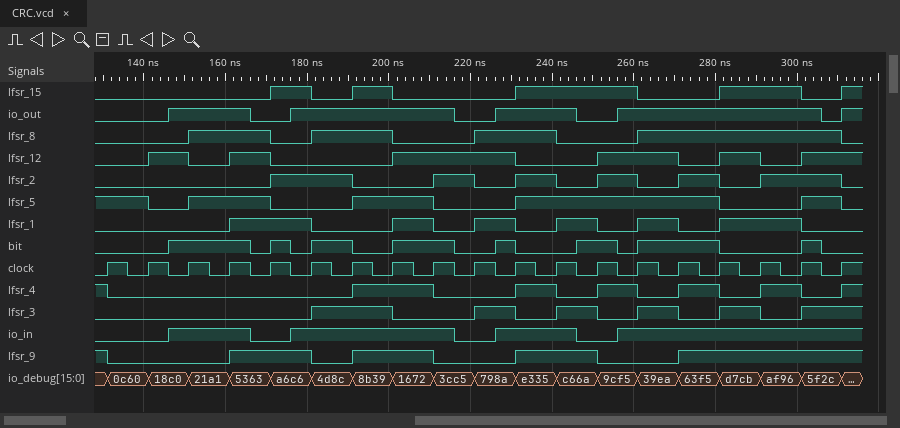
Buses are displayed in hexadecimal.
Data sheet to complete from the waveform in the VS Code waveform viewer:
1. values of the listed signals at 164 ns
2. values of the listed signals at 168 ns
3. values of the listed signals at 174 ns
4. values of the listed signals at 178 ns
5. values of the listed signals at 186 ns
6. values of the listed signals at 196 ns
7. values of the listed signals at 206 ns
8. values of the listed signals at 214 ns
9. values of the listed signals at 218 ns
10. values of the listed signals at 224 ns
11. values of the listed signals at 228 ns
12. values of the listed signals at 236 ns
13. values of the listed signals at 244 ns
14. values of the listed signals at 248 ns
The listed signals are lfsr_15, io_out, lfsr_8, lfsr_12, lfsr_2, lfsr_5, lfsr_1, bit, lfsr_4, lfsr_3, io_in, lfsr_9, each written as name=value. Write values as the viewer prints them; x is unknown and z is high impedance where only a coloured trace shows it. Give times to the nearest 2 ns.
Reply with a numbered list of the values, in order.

1. lfsr_15=0, io_out=1, lfsr_8=1, lfsr_12=1, lfsr_2=0, lfsr_5=1, lfsr_1=1, bit=1, lfsr_4=0, lfsr_3=0, io_in=1, lfsr_9=1
2. lfsr_15=0, io_out=0, lfsr_8=1, lfsr_12=1, lfsr_2=0, lfsr_5=1, lfsr_1=1, bit=0, lfsr_4=0, lfsr_3=0, io_in=0, lfsr_9=1
3. lfsr_15=1, io_out=0, lfsr_8=0, lfsr_12=0, lfsr_2=1, lfsr_5=0, lfsr_1=1, bit=1, lfsr_4=0, lfsr_3=0, io_in=0, lfsr_9=1
4. lfsr_15=1, io_out=1, lfsr_8=0, lfsr_12=0, lfsr_2=1, lfsr_5=0, lfsr_1=1, bit=0, lfsr_4=0, lfsr_3=0, io_in=1, lfsr_9=1
5. lfsr_15=0, io_out=1, lfsr_8=1, lfsr_12=0, lfsr_2=1, lfsr_5=0, lfsr_1=0, bit=1, lfsr_4=0, lfsr_3=1, io_in=1, lfsr_9=0
6. lfsr_15=1, io_out=1, lfsr_8=1, lfsr_12=0, lfsr_2=0, lfsr_5=1, lfsr_1=0, bit=0, lfsr_4=1, lfsr_3=1, io_in=1, lfsr_9=1
7. lfsr_15=0, io_out=1, lfsr_8=0, lfsr_12=1, lfsr_2=0, lfsr_5=1, lfsr_1=1, bit=1, lfsr_4=1, lfsr_3=0, io_in=1, lfsr_9=1
8. lfsr_15=0, io_out=1, lfsr_8=0, lfsr_12=1, lfsr_2=1, lfsr_5=0, lfsr_1=0, bit=1, lfsr_4=0, lfsr_3=0, io_in=1, lfsr_9=0
9. lfsr_15=0, io_out=0, lfsr_8=0, lfsr_12=1, lfsr_2=1, lfsr_5=0, lfsr_1=0, bit=0, lfsr_4=0, lfsr_3=0, io_in=0, lfsr_9=0
10. lfsr_15=0, io_out=0, lfsr_8=1, lfsr_12=1, lfsr_2=0, lfsr_5=0, lfsr_1=1, bit=0, lfsr_4=0, lfsr_3=1, io_in=0, lfsr_9=0
11. lfsr_15=0, io_out=1, lfsr_8=1, lfsr_12=1, lfsr_2=0, lfsr_5=0, lfsr_1=1, bit=1, lfsr_4=0, lfsr_3=1, io_in=1, lfsr_9=0
12. lfsr_15=1, io_out=1, lfsr_8=1, lfsr_12=0, lfsr_2=1, lfsr_5=1, lfsr_1=0, bit=0, lfsr_4=1, lfsr_3=0, io_in=1, lfsr_9=1
13. lfsr_15=1, io_out=1, lfsr_8=0, lfsr_12=0, lfsr_2=0, lfsr_5=1, lfsr_1=1, bit=0, lfsr_4=0, lfsr_3=1, io_in=1, lfsr_9=1
14. lfsr_15=1, io_out=0, lfsr_8=0, lfsr_12=0, lfsr_2=0, lfsr_5=1, lfsr_1=1, bit=1, lfsr_4=0, lfsr_3=1, io_in=0, lfsr_9=1
